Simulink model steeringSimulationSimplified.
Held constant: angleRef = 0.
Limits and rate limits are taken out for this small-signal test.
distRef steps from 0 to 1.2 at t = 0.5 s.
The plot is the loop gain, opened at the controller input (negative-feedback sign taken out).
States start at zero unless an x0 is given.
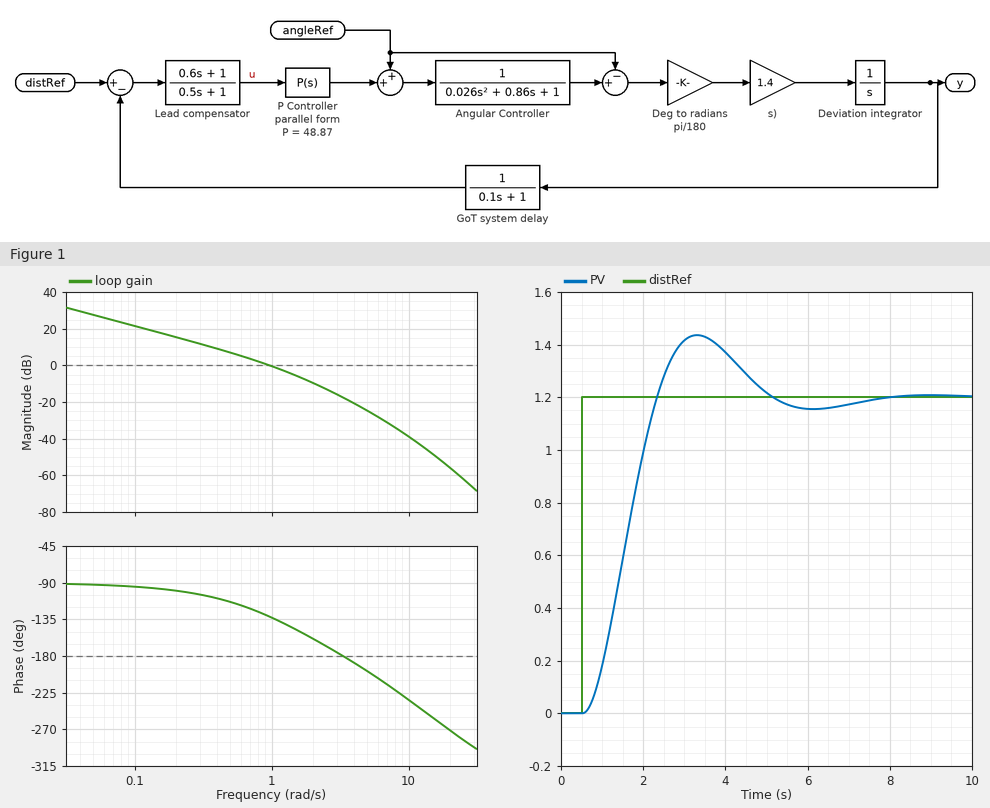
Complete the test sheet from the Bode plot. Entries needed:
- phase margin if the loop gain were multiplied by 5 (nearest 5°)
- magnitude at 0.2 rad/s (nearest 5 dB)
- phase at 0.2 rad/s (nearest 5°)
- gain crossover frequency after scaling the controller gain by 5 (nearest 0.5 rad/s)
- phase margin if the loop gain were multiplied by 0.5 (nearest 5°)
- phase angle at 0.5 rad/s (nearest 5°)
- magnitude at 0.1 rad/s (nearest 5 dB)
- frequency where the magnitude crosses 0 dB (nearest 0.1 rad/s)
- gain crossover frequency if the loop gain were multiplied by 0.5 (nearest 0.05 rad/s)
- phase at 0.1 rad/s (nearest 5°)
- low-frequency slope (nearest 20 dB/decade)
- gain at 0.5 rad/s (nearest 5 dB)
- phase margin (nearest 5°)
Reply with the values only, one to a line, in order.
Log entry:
10°
15 dB
-100°
2.5 rad/s
65°
-115°
20 dB
1.0 rad/s
0.55 rad/s
-95°
-20 dB/decade
5 dB
50°
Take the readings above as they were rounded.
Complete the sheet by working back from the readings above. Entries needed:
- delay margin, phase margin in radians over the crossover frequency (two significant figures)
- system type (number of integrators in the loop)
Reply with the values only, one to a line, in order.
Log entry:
0.87 s
1
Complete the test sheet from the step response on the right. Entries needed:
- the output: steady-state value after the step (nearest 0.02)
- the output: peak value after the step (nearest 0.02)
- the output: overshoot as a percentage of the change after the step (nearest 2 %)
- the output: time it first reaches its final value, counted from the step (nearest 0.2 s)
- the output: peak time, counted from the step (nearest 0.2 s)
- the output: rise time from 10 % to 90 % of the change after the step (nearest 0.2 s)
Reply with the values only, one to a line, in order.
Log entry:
1.20
1.44
20 %
1.8 s
2.8 s
1.2 s
